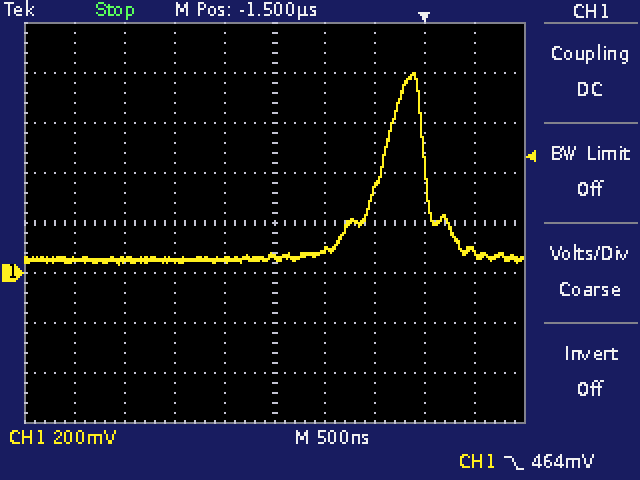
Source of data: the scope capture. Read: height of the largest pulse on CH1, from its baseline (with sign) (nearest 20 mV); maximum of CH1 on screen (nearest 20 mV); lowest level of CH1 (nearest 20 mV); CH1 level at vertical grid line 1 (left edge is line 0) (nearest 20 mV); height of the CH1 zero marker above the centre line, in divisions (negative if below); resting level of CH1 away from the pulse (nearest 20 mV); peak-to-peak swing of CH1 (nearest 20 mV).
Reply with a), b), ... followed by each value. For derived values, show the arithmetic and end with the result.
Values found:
a) 800 mV − (60 mV) = +740 mV
b) 800 mV
c) 40 mV
d) 60 mV
e) -1.0 div
f) 60 mV
g) 800 mV − (40 mV) = 760 mV
